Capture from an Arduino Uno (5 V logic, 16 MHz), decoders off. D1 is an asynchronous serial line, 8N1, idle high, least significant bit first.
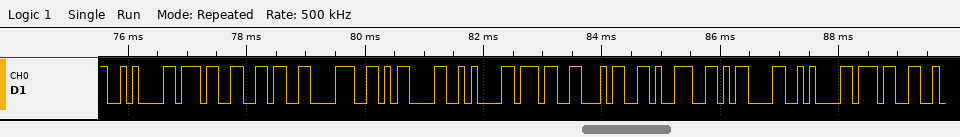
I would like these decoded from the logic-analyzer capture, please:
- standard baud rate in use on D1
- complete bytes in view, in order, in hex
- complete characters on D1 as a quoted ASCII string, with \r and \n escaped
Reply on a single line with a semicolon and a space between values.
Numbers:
9600 baud; 0x0A 0x37 0x36 0x38 0x0D 0x0A 0x37 0x34 0x39 0x0D 0x0A 0x37; "\n768\r\n749\r\n7"
